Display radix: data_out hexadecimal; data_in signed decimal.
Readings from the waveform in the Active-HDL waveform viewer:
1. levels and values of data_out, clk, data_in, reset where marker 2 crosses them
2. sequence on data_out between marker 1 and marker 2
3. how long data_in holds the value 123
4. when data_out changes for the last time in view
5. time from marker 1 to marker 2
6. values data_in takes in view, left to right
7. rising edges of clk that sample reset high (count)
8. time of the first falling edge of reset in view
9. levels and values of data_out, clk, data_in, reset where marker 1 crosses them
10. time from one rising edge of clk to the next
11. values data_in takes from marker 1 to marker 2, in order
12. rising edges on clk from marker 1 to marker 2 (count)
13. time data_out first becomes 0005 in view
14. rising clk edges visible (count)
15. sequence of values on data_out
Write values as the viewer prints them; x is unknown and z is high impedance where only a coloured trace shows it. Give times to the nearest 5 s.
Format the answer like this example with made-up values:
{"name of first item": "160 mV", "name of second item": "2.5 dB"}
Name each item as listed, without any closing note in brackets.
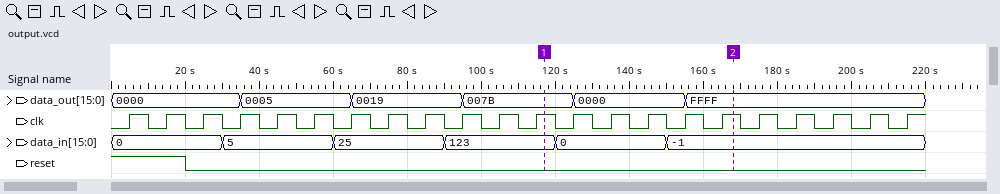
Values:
{"levels and values of data_out, clk, data_in, reset where marker 2 crosses them": "data_out=FFFF, clk=1, data_in=-1, reset=0", "sequence on data_out between marker 1 and marker 2": "007B, 0000, FFFF", "how long data_in holds the value 123": "30 s", "when data_out changes for the last time in view": "155 s", "time from marker 1 to marker 2": "50 s", "values data_in takes in view, left to right": "0, 5, 25, 123, 0, -1", "rising edges of clk that sample reset high": "2", "time of the first falling edge of reset in view": "20 s", "levels and values of data_out, clk, data_in, reset where marker 1 crosses them": "data_out=007B, clk=1, data_in=123, reset=0", "time from one rising edge of clk to the next": "10 s", "values data_in takes from marker 1 to marker 2, in order": "123, 0, -1", "rising edges on clk from marker 1 to marker 2": "5", "time data_out first becomes 0005 in view": "35 s", "rising clk edges visible": "22", "sequence of values on data_out": "0000, 0005, 0019, 007B, 0000, FFFF"}
